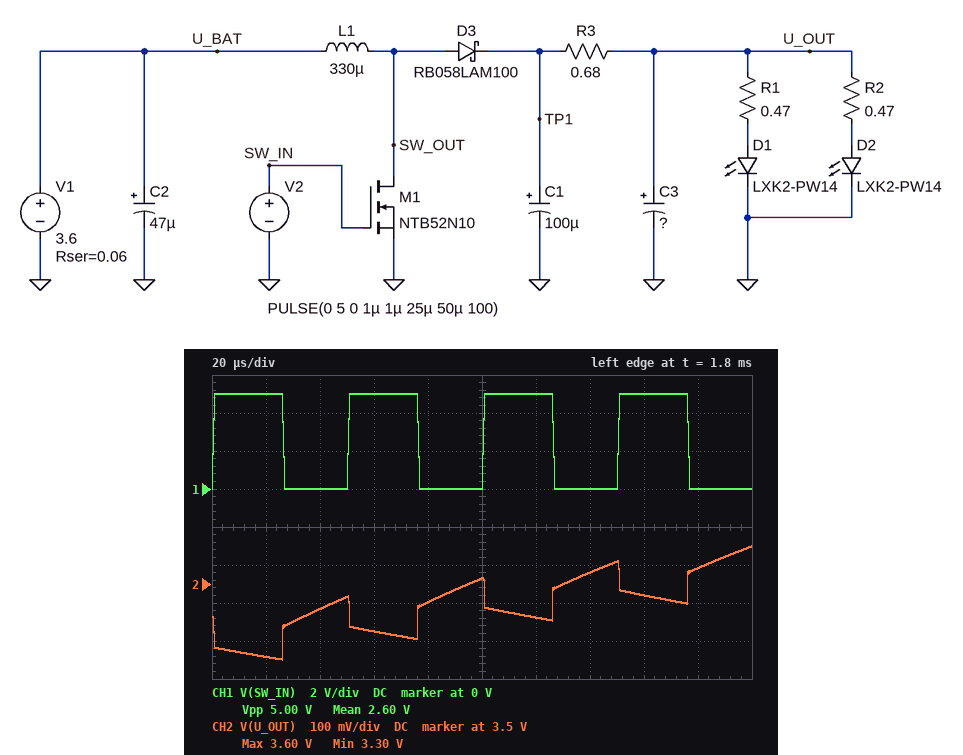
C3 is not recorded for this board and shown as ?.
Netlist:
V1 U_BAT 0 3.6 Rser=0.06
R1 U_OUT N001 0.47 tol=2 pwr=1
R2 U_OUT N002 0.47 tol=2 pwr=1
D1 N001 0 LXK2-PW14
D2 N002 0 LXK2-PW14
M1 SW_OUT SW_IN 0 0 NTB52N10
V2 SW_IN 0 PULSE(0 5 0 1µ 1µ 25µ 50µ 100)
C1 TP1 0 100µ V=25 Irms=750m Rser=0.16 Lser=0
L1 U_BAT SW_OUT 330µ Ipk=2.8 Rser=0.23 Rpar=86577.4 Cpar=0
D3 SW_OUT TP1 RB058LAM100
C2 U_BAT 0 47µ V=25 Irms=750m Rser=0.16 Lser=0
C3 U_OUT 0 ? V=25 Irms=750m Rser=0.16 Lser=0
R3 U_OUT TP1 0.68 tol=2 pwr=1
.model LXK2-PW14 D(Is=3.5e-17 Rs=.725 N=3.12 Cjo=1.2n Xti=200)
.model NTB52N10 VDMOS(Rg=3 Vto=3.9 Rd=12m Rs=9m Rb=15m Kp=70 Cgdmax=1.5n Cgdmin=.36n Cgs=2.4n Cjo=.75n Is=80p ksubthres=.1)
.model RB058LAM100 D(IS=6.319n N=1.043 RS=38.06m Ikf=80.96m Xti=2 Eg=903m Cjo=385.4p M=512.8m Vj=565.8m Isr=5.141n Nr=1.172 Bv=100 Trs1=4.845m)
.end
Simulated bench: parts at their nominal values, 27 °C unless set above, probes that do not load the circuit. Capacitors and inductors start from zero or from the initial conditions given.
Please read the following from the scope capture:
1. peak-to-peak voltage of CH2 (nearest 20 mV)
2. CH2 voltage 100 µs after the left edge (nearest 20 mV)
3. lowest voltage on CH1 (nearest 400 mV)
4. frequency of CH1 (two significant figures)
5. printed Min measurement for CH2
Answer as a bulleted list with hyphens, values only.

- 300 mV
- 3.52 V
- 0 V
- 20 kHz
- 3.30 V
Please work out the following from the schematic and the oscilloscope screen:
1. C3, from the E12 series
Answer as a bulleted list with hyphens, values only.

- 820 µF
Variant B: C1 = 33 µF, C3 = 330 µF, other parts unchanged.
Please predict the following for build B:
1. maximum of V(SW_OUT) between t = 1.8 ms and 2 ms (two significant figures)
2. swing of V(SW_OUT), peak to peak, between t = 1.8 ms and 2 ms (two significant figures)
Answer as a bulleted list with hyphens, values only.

- 6.1 V
- 6.0 V
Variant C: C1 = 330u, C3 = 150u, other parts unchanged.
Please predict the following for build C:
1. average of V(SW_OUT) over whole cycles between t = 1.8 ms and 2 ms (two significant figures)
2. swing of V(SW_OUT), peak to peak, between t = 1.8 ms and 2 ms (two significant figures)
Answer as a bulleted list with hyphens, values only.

- 3.0 V
- 5.9 V
